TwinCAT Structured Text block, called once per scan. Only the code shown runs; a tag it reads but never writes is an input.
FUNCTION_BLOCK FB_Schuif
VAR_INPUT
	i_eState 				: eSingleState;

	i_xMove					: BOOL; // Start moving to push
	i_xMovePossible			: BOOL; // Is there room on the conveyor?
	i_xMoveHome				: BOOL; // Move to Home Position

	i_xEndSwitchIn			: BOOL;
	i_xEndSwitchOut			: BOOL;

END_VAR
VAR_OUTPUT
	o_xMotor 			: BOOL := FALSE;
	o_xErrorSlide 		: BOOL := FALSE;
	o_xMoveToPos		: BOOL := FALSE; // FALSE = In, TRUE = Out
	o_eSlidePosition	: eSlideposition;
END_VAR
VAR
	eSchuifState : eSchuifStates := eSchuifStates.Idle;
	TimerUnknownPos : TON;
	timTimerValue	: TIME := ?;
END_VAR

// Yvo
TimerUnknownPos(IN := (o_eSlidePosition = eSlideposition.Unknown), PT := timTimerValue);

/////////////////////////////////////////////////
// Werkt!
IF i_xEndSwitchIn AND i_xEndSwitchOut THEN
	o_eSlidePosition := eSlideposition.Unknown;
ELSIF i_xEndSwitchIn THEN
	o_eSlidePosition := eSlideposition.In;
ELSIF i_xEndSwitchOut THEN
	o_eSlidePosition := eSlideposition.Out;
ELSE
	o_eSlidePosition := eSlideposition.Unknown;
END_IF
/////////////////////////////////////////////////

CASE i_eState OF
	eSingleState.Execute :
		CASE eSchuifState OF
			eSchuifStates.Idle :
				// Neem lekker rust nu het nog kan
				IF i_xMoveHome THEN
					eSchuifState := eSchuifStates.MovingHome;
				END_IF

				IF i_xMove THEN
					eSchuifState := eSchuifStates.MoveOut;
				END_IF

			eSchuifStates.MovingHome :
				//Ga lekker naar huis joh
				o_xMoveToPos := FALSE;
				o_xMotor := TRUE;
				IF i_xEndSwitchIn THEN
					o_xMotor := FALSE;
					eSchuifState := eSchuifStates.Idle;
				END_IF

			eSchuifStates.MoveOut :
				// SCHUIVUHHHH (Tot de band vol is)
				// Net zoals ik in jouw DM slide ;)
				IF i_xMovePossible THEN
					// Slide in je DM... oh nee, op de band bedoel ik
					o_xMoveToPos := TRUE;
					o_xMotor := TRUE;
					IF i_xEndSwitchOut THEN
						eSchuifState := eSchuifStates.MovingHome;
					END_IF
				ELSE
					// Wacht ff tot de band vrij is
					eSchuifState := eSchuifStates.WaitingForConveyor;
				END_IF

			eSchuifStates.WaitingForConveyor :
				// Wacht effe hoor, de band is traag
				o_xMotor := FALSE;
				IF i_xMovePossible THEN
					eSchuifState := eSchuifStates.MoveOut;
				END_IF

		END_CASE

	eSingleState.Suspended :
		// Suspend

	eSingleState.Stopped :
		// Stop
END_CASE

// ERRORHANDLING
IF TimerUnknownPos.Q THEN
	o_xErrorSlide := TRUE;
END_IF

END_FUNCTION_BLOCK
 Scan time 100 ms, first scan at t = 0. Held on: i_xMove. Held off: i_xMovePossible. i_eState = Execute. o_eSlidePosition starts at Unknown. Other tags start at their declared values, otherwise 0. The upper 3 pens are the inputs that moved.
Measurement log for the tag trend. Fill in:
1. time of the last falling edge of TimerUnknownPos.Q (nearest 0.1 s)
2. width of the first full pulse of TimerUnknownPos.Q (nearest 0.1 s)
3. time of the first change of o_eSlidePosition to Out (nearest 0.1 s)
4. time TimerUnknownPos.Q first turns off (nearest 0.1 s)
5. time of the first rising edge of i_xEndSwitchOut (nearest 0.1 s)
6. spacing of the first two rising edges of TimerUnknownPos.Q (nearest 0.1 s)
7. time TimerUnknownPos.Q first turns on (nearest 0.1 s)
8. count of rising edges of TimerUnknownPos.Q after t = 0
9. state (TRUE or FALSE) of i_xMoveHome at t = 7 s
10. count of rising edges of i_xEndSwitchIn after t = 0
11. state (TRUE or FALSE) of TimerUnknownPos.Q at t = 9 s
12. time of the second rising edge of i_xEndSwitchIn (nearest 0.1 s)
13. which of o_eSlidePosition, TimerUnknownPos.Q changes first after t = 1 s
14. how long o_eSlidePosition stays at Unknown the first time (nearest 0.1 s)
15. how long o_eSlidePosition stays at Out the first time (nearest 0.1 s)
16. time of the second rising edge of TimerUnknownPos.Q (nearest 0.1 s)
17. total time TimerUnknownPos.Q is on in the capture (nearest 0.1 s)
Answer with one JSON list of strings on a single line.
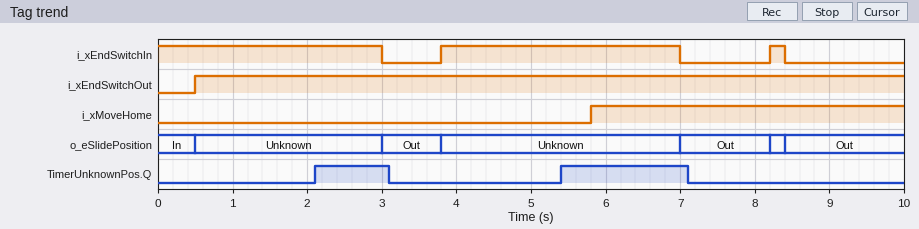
["7.1 s", "1.0 s", "3.0 s", "3.1 s", "0.5 s", "3.3 s", "2.1 s", "2", "TRUE", "2", "FALSE", "8.2 s", "TimerUnknownPos.Q", "2.5 s", "0.8 s", "5.4 s", "2.7 s"]
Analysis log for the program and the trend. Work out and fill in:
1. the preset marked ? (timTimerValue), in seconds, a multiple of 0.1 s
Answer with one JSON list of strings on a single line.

["1.5 s"]
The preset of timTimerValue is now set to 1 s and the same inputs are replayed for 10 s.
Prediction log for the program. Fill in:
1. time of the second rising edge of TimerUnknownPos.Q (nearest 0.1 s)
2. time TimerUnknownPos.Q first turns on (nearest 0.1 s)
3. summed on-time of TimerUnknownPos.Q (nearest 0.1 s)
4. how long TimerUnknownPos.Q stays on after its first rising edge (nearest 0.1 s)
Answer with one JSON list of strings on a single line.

["4.9 s", "1.6 s", "3.7 s", "1.5 s"]
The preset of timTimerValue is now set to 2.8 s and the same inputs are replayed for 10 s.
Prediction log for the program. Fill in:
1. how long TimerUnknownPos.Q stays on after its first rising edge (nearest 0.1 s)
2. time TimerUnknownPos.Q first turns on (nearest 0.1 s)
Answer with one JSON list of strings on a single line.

["0.4 s", "6.7 s"]
